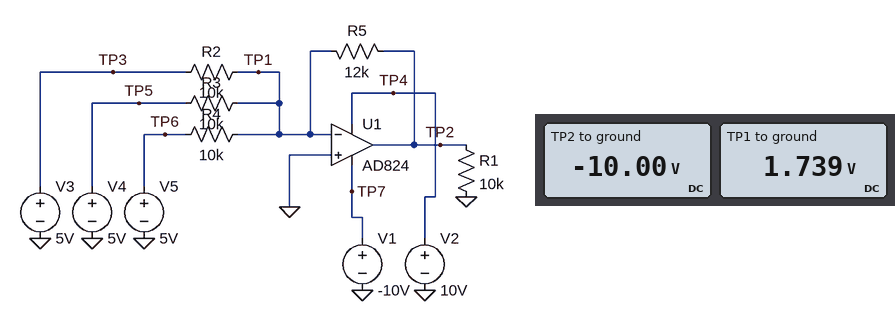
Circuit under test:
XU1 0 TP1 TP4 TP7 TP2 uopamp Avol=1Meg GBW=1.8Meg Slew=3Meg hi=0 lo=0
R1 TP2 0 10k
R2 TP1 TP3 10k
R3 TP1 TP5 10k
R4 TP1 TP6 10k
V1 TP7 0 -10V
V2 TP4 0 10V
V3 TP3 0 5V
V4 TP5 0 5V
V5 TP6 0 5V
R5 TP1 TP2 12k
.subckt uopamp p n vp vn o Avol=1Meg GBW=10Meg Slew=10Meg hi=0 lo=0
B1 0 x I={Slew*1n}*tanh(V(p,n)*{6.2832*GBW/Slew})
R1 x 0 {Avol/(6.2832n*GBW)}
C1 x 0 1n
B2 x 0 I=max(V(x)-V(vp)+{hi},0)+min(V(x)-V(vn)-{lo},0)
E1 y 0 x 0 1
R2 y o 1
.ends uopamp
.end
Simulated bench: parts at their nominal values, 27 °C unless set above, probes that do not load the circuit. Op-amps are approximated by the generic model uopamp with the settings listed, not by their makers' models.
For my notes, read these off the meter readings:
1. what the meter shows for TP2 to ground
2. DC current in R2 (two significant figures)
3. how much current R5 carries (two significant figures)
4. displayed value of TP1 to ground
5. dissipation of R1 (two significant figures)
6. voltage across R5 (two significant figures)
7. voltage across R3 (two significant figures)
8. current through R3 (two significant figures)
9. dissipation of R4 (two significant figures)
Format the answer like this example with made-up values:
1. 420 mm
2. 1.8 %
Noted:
1. -10.00 V
2. 330 µA
3. 980 µA
4. 1.739 V
5. 10 mW
6. 12 V
7. 3.3 V
8. 330 µA
9. 1.1 mW
